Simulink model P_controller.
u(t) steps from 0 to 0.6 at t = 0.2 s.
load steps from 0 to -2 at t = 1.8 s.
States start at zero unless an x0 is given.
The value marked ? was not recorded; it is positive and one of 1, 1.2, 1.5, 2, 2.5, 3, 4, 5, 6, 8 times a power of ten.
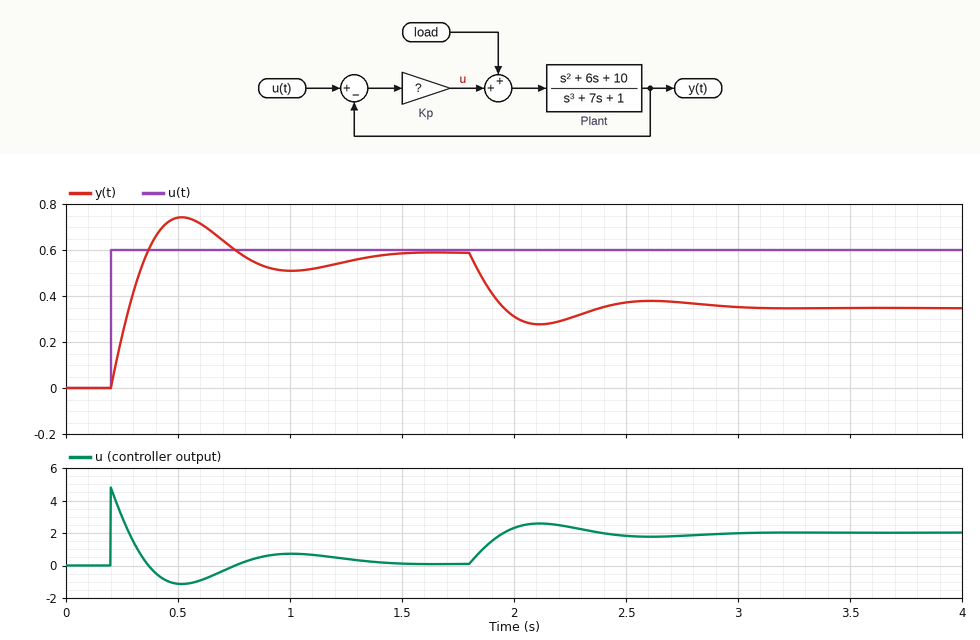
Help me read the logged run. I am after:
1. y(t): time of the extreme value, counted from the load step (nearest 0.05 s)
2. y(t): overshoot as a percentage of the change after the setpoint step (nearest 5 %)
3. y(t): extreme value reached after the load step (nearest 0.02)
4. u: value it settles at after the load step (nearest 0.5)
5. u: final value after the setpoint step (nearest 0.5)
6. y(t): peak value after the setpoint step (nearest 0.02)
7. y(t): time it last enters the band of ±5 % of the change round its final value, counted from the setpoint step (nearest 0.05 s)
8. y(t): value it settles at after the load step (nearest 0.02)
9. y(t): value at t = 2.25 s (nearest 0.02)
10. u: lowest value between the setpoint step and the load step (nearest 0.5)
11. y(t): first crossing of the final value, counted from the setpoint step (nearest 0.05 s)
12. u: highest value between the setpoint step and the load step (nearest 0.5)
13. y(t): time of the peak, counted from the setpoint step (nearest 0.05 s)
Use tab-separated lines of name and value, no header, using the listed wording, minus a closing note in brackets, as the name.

y(t): time of the extreme value, counted from the load step	0.30 s
y(t): overshoot as a percentage of the change after the setpoint step	25 %
y(t): extreme value reached after the load step	0.28
u: value it settles at after the load step	2.0
u: final value after the setpoint step	0.0
y(t): peak value after the setpoint step	0.74
y(t): time it last enters the band of ±5 % of the change round its final value, counted from the setpoint step	1.10 s
y(t): value it settles at after the load step	0.34
y(t): value at t = 2.25 s	0.30
u: lowest value between the setpoint step and the load step	-1.0
y(t): first crossing of the final value, counted from the setpoint step	0.15 s
u: highest value between the setpoint step and the load step	5.0
y(t): time of the peak, counted from the setpoint step	0.30 s
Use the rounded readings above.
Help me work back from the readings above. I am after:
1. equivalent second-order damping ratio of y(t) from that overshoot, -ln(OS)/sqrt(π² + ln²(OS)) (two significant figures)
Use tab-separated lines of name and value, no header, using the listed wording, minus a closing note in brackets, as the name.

equivalent second-order damping ratio of y(t) from that overshoot, -ln(OS)/sqrt(π² + ln²(OS))	0.40
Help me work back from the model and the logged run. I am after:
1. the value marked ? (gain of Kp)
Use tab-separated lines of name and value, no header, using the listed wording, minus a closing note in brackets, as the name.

the value marked ?	8
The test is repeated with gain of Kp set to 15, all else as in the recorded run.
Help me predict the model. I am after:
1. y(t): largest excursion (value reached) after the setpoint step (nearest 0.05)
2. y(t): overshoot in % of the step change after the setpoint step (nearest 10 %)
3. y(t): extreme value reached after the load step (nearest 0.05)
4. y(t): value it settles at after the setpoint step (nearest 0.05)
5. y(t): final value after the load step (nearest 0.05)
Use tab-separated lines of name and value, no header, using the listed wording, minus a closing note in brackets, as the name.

y(t): largest excursion (value reached) after the setpoint step	0.70
y(t): overshoot in % of the step change after the setpoint step	20 %
y(t): extreme value reached after the load step	0.45
y(t): value it settles at after the setpoint step	0.60
y(t): final value after the load step	0.45
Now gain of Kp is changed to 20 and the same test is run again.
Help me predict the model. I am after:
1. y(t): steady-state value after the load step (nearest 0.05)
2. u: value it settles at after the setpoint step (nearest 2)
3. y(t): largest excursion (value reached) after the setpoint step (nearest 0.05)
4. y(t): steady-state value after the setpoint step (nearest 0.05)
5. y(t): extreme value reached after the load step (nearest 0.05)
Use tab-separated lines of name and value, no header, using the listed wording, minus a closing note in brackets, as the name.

y(t): steady-state value after the load step	0.50
u: value it settles at after the setpoint step	0
y(t): largest excursion (value reached) after the setpoint step	0.70
y(t): steady-state value after the setpoint step	0.60
y(t): extreme value reached after the load step	0.50
